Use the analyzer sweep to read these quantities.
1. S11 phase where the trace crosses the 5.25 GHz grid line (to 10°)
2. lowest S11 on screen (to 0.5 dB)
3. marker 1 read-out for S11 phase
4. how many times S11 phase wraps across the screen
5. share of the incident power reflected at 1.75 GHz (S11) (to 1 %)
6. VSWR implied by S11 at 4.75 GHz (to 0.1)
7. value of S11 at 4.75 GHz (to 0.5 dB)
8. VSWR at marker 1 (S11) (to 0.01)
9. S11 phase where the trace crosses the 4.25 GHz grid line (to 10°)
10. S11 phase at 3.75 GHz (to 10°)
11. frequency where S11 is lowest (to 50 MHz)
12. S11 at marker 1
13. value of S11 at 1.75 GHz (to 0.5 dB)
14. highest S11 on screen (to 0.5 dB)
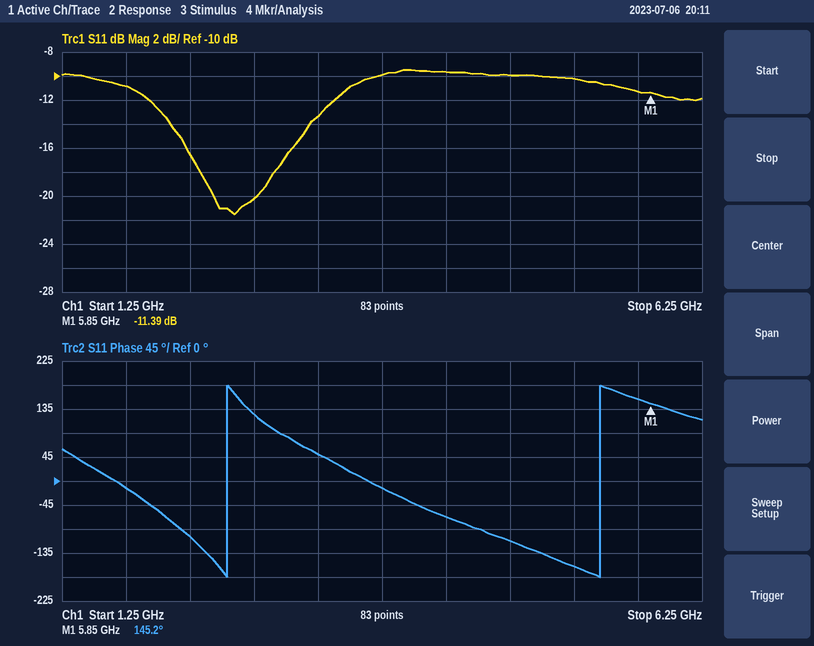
-160°
-21.5 dB
145.2°
2
8 %
1.9
-10.0 dB
1.74
-70°
-10°
2.60 GHz
-11.39 dB
-11.0 dB
-9.5 dB
